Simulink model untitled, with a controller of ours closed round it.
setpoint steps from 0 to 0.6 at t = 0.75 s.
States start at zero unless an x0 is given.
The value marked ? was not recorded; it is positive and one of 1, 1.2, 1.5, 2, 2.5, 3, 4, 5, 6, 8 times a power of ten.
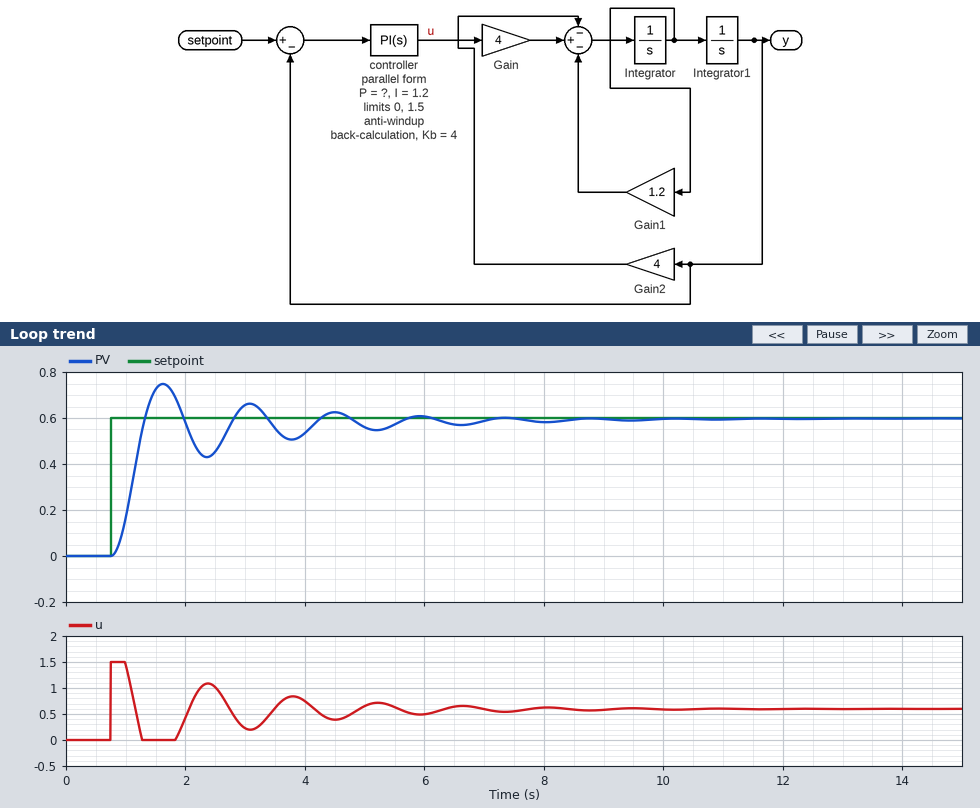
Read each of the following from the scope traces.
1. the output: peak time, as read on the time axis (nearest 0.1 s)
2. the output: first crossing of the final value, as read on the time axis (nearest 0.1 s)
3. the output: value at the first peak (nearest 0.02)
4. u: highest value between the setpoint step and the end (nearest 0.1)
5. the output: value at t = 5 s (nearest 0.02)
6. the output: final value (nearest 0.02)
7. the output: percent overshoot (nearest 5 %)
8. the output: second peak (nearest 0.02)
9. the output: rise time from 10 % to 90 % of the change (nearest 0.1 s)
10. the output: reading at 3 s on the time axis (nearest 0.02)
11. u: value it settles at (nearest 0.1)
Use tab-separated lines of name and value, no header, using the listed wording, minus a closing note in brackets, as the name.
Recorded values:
the output: peak time, as read on the time axis	1.6 s
the output: first crossing of the final value, as read on the time axis	1.3 s
the output: value at the first peak	0.74
u: highest value between the setpoint step and the end	1.5
the output: value at t = 5 s	0.56
the output: final value	0.60
the output: percent overshoot	25 %
the output: second peak	0.66
the output: rise time from 10 % to 90 % of the change	0.4 s
the output: reading at 3 s on the time axis	0.66
u: value it settles at	0.6
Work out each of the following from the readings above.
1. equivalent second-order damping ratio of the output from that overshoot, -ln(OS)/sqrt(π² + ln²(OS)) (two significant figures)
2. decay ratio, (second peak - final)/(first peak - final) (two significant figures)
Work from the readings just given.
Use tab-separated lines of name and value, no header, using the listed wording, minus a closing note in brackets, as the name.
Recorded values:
equivalent second-order damping ratio of the output from that overshoot, -ln(OS)/sqrt(π² + ln²(OS))	0.40
decay ratio, (second peak - final)/(first peak - final)	0.43
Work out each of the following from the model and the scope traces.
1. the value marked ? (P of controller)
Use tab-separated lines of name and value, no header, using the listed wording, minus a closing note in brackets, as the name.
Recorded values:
the value marked ?	4
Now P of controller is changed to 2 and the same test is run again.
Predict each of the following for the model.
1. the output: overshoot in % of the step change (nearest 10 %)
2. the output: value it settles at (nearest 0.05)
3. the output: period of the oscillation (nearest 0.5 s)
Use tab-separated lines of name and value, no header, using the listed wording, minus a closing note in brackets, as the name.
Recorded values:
the output: overshoot in % of the step change	30 %
the output: value it settles at	0.60
the output: period of the oscillation	2.0 s
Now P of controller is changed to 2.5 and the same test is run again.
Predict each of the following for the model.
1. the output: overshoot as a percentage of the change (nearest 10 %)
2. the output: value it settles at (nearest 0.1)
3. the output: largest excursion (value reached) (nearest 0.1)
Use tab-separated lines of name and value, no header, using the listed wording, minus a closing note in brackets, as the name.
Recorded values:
the output: overshoot as a percentage of the change	30 %
the output: value it settles at	0.6
the output: largest excursion (value reached)	0.8
